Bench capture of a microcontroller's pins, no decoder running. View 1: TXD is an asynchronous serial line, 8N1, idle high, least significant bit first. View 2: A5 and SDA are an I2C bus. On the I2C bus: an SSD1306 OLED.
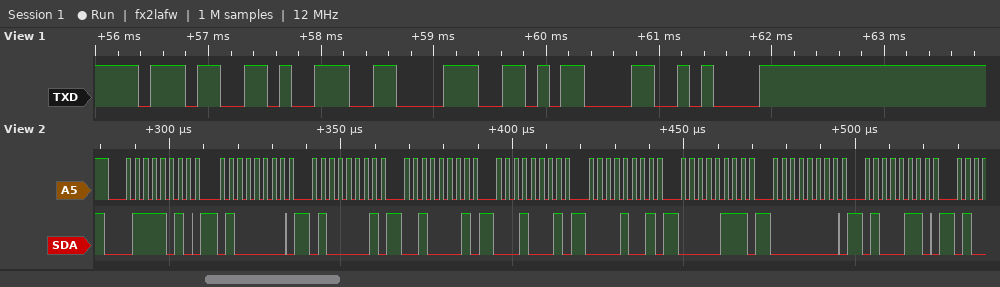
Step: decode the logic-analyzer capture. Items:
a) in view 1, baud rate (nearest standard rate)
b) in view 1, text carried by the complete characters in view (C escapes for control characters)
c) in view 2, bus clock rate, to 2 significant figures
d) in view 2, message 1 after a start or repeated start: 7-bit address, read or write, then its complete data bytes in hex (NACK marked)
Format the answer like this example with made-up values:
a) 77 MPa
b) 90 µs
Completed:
a) 9600 baud
b) "798\r\n"
c) 400 kHz
d) 0x3D write: 40 41 21 11 09 07 00 46
